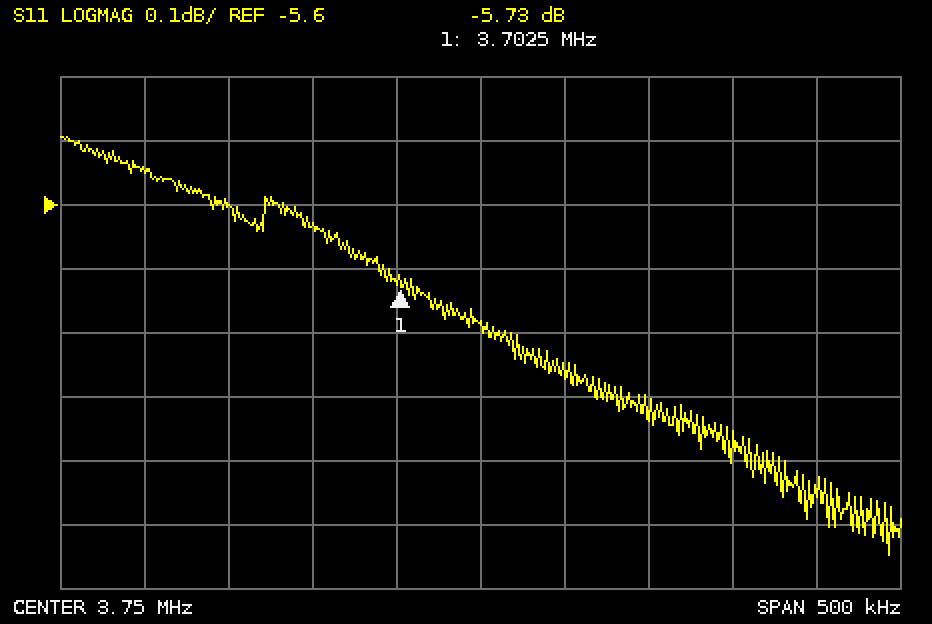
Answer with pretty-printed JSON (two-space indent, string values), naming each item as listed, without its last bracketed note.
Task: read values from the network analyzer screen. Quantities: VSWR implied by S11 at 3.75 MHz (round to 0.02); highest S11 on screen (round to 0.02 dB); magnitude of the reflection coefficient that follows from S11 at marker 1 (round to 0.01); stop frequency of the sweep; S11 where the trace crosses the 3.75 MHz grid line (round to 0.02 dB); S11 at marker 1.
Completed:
{
  "VSWR implied by S11 at 3.75 MHz": "3.12",
  "highest S11 on screen": "-5.50 dB",
  "magnitude of the reflection coefficient that follows from S11 at marker 1": "0.52",
  "stop frequency of the sweep": "4 MHz",
  "S11 where the trace crosses the 3.75 MHz grid line": "-5.78 dB",
  "S11 at marker 1": "-5.73 dB"
}
